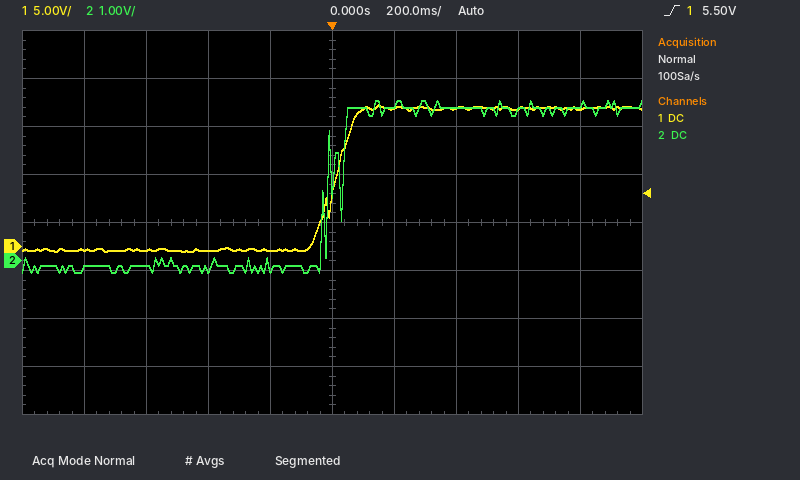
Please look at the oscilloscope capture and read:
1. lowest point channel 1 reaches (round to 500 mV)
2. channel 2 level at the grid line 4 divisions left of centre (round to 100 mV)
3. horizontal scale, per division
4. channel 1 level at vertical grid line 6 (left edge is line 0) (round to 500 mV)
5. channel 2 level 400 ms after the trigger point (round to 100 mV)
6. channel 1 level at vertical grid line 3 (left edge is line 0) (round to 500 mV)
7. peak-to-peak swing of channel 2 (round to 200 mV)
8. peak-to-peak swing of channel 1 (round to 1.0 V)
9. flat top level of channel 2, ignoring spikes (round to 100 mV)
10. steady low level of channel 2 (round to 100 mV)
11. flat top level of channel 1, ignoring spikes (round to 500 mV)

-500 mV
-200 mV
200 ms
14.5 V
3.2 V
-500 mV
3.6 V
15.0 V
3.2 V
-100 mV
14.5 V
